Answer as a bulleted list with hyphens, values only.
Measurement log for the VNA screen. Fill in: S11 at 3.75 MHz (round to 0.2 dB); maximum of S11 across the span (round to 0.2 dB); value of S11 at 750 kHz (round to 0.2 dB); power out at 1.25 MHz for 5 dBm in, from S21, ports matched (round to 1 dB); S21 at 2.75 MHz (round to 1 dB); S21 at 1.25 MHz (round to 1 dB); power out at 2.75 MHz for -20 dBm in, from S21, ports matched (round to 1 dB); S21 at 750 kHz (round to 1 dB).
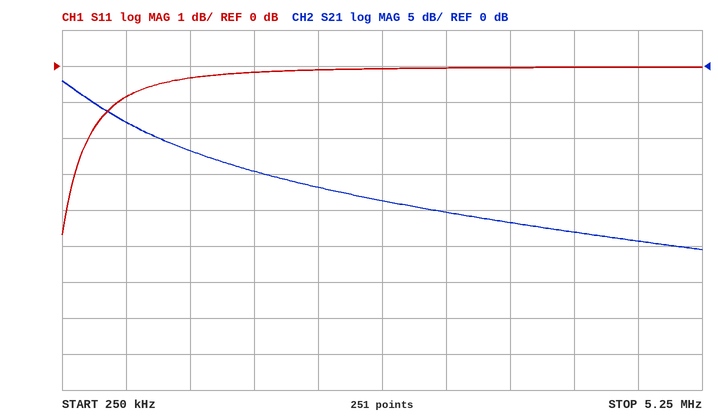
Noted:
- 0.0 dB
- 0.0 dB
- -0.8 dB
- -7 dBm
- -19 dB
- -12 dB
- -39 dBm
- -8 dB
